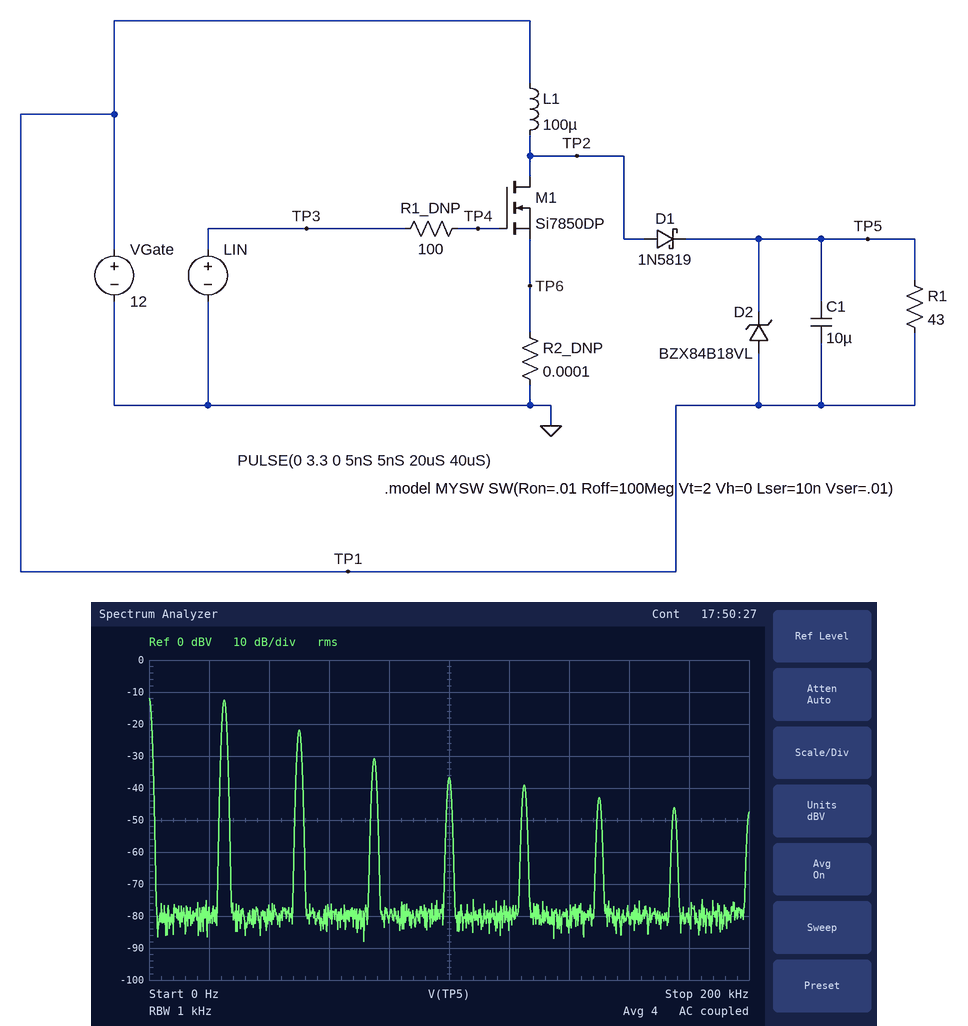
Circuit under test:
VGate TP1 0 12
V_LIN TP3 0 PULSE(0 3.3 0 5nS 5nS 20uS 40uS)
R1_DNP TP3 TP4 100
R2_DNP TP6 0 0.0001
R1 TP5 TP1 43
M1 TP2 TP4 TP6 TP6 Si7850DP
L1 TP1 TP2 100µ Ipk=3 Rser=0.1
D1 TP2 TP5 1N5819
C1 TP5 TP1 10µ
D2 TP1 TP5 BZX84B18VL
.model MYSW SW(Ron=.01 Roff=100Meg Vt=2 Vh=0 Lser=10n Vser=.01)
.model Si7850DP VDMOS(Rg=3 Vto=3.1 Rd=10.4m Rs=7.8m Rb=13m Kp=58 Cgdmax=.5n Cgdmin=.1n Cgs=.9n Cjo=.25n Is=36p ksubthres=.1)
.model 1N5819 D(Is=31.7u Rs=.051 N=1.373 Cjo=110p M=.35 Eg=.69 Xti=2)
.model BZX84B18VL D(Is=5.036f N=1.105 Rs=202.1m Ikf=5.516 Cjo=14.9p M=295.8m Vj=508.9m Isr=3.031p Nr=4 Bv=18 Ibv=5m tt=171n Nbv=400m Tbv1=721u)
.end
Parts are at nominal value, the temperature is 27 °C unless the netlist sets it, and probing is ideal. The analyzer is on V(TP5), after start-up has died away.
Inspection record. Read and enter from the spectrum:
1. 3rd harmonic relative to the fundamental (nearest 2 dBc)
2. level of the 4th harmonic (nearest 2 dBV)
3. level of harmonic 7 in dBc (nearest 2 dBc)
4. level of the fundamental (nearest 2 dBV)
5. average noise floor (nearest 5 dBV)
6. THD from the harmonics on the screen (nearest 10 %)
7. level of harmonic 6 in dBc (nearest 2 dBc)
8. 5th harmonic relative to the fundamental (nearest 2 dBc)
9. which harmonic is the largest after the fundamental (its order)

-18 dBc
-36 dBV
-34 dBc
-12 dBV
-80 dBV
40 %
-30 dBc
-26 dBc
2
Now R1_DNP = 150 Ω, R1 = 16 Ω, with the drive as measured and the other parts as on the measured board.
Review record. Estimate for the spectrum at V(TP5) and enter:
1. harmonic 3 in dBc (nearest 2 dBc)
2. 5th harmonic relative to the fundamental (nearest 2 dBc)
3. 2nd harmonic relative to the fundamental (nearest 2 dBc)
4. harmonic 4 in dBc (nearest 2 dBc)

-20 dBc
-30 dBc
-14 dBc
-26 dBc
